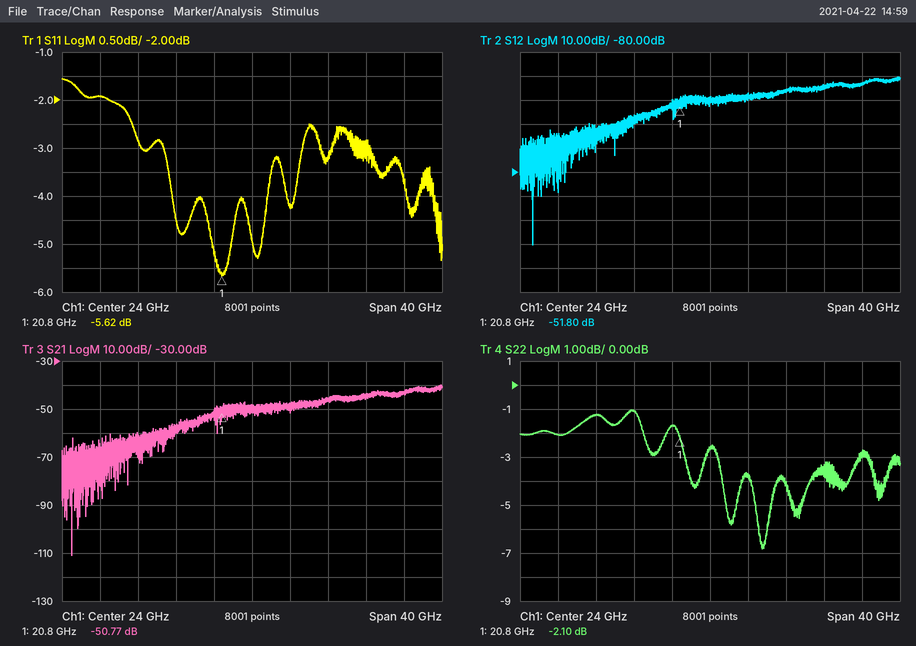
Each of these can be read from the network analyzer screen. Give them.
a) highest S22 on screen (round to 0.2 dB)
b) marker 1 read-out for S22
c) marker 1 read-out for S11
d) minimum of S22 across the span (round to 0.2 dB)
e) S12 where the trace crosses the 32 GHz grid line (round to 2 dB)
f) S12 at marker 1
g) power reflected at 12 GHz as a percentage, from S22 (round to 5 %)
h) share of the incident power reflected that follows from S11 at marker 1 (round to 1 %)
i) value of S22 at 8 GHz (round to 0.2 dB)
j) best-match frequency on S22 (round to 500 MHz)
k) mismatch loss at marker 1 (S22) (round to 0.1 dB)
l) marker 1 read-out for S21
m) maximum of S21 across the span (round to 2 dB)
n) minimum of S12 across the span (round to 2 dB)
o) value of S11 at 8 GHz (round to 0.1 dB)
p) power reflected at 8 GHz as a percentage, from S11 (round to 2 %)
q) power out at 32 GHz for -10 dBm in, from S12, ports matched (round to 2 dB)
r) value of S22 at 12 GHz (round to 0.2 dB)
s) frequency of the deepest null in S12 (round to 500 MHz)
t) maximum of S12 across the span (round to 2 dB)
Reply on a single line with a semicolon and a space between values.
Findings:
-1.0 dB; -2.10 dB; -5.62 dB; -6.8 dB; -46 dB; -51.80 dB; 75 %; 27 %; -2.0 dB; 29.5 GHz; 4.2 dB; -50.77 dB; -40 dB; -110 dB; -1.9 dB; 64 %; -56 dBm; -1.2 dB; 5.5 GHz; -40 dB
